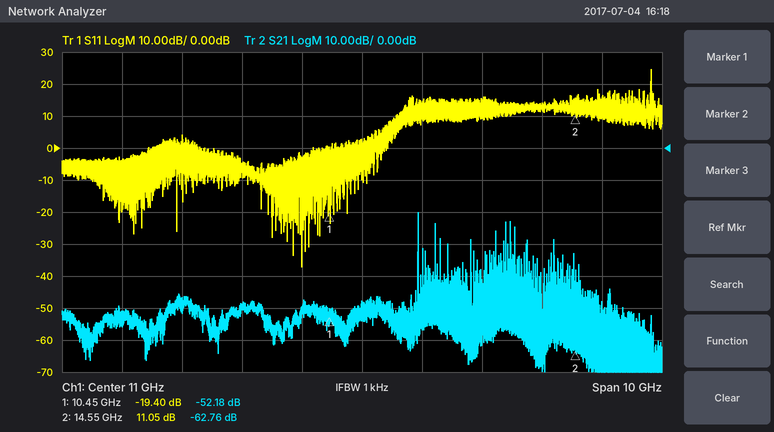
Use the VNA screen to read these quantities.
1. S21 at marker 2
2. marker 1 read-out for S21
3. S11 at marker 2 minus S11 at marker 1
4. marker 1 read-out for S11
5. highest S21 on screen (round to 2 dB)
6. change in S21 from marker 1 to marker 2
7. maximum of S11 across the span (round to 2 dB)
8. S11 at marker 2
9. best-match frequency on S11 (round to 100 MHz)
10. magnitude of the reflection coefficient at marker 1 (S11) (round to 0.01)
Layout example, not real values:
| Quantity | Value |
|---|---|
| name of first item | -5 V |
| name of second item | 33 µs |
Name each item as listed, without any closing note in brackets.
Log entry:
| Quantity | Value |
|---|---|
| S21 at marker 2 | -62.76 dB |
| marker 1 read-out for S21 | -52.18 dB |
| S11 at marker 2 minus S11 at marker 1 | 30.45 dB |
| marker 1 read-out for S11 | -19.40 dB |
| highest S21 on screen | -20 dB |
| change in S21 from marker 1 to marker 2 | -10.58 dB |
| maximum of S11 across the span | 24 dB |
| S11 at marker 2 | 11.05 dB |
| best-match frequency on S11 | 10.0 GHz |
| magnitude of the reflection coefficient at marker 1 (S11) | 0.11 |
